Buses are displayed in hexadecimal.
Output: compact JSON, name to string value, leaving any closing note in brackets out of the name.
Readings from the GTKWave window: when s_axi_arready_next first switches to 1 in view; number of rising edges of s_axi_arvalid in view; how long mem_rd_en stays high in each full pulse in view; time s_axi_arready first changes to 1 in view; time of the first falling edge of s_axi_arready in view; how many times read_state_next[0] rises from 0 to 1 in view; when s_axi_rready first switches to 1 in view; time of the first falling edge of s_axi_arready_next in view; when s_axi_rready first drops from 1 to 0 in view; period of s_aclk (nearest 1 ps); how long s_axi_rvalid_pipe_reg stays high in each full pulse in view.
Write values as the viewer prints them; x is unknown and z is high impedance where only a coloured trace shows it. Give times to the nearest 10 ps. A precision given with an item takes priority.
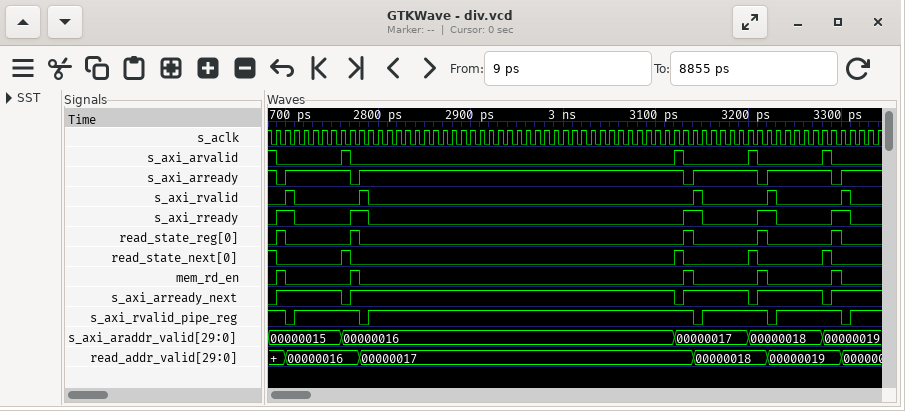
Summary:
{"when s_axi_arready_next first switches to 1 in view": "2690 ps", "number of rising edges of s_axi_arvalid in view": "4", "how long mem_rd_en stays high in each full pulse in view": "10 ps, 10 ps, 10 ps, 10 ps, 10 ps", "time s_axi_arready first changes to 1 in view": "2700 ps", "time of the first falling edge of s_axi_arready in view": "2690 ps", "how many times read_state_next[0] rises from 0 to 1 in view": "4", "when s_axi_rready first switches to 1 in view": "2690 ps", "time of the first falling edge of s_axi_arready_next in view": "2760 ps", "when s_axi_rready first drops from 1 to 0 in view": "2710 ps", "period of s_aclk": "10 ps", "how long s_axi_rvalid_pipe_reg stays high in each full pulse in view": "70 ps, 350 ps, 70 ps, 70 ps"}
